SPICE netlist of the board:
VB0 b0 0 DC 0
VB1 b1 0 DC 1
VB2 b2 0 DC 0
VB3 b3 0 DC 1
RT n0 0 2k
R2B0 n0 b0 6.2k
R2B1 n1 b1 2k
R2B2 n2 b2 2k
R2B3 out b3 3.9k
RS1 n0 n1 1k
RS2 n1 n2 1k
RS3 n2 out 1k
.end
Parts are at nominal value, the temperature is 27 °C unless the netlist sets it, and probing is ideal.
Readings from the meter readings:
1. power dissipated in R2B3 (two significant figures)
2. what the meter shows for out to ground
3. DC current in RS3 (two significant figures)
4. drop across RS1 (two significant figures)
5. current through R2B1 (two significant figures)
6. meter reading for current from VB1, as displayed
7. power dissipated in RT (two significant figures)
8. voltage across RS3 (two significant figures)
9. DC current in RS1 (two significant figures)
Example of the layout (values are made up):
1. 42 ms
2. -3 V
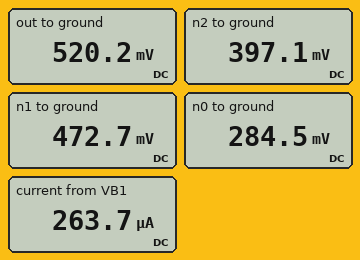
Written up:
1. 59 µW
2. 520.2 mV
3. 120 µA
4. 190 mV
5. 260 µA
6. 263.7 µA
7. 40 µW
8. 120 mV
9. 190 µA
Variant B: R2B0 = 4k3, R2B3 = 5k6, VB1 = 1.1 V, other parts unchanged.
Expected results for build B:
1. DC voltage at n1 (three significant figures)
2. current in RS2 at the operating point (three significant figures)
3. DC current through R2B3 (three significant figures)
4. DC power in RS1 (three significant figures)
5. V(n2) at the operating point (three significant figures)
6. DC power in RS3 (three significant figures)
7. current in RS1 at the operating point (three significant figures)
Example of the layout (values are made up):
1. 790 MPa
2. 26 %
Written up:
1. 487 mV
2. 100 µA
3. 92.9 µA
4. 42.4 µW
5. 387 mV
6. 8.63 µW
7. 206 µA
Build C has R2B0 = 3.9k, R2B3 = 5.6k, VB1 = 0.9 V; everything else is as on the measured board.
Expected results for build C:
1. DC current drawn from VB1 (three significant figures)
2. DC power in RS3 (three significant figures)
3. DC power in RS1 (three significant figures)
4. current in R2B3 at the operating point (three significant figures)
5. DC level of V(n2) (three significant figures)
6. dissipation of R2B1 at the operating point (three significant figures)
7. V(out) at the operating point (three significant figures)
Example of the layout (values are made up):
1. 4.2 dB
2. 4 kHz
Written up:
1. 246 µA
2. 10.0 µW
3. 31.0 µW
4. 100 µA
5. 339 mV
6. 121 µW
7. 439 mV
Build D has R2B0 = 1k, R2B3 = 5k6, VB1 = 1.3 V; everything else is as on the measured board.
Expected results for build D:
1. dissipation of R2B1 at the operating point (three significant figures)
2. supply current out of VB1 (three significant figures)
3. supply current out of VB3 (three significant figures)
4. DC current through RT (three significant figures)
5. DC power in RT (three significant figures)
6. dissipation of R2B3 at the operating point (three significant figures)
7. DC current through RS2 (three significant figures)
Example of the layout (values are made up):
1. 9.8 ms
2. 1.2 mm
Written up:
1. 323 µW
2. 402 µA
3. 92.1 µA
4. 99.3 µA
5. 19.7 µW
6. 47.5 µW
7. 104 µA
